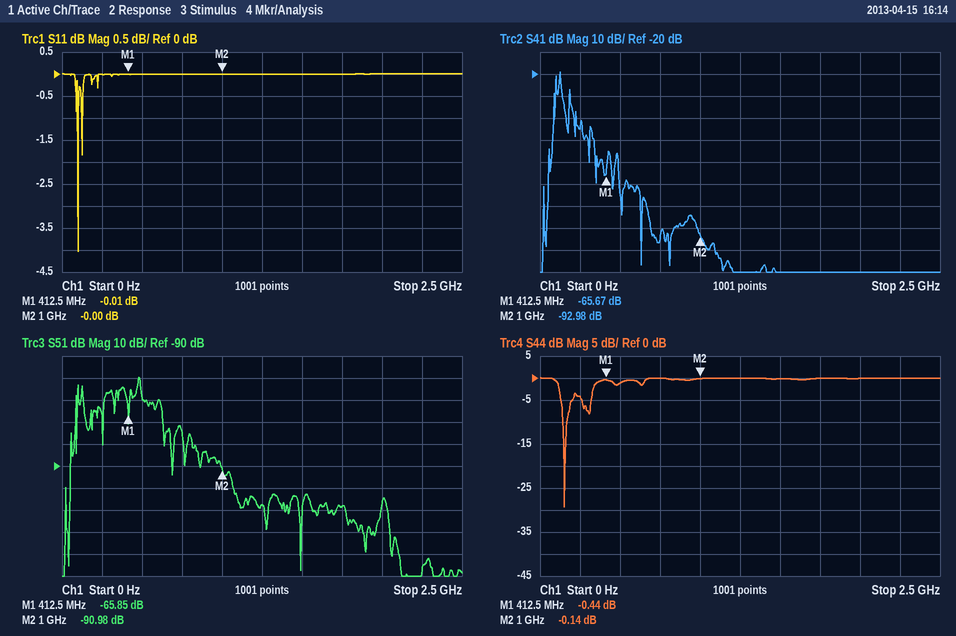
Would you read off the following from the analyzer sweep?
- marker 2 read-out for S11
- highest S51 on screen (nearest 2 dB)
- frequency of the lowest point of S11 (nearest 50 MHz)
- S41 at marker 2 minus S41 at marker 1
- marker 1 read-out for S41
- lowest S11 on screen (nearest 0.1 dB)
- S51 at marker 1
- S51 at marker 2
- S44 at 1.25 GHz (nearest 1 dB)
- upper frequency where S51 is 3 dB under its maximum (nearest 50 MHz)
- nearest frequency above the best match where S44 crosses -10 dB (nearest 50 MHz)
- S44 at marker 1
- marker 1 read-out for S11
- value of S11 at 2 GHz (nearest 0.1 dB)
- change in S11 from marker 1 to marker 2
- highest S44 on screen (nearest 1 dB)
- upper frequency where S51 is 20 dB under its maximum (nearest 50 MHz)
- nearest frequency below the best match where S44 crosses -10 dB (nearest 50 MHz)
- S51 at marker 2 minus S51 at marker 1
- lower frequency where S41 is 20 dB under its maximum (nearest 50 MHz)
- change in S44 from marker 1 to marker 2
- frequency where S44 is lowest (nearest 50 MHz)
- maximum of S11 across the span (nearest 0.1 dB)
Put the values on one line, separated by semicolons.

-0.00 dB; -50 dB; 100 MHz; -27.31 dB; -65.67 dB; -4.0 dB; -65.85 dB; -90.98 dB; 0 dB; 500 MHz; 150 MHz; -0.44 dB; -0.01 dB; 0.0 dB; 0.01 dB; 0 dB; 650 MHz; 150 MHz; -25.13 dB; 100 MHz; 0.30 dB; 150 MHz; 0.0 dB
